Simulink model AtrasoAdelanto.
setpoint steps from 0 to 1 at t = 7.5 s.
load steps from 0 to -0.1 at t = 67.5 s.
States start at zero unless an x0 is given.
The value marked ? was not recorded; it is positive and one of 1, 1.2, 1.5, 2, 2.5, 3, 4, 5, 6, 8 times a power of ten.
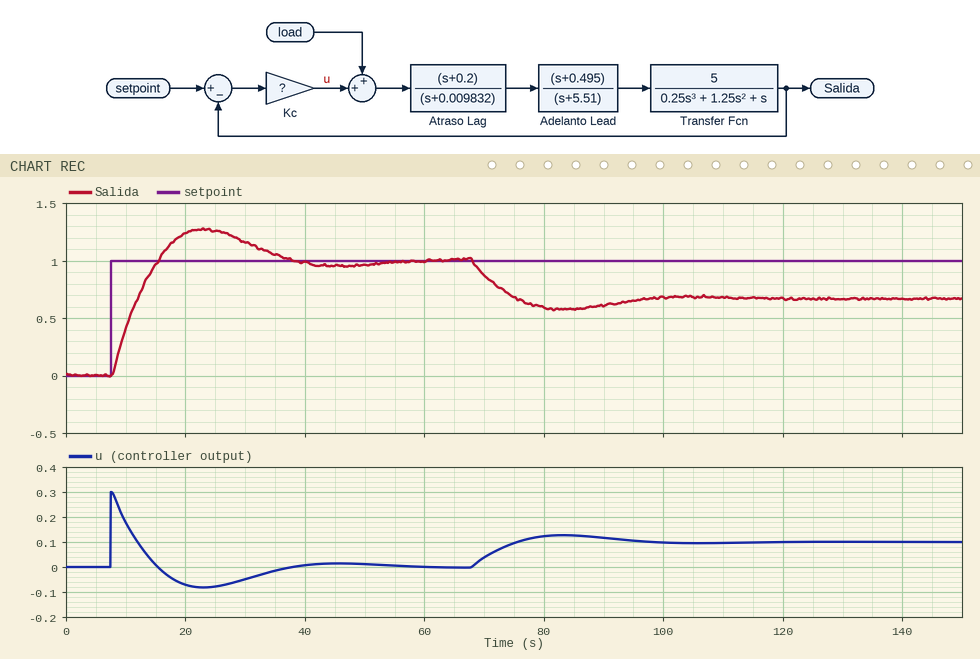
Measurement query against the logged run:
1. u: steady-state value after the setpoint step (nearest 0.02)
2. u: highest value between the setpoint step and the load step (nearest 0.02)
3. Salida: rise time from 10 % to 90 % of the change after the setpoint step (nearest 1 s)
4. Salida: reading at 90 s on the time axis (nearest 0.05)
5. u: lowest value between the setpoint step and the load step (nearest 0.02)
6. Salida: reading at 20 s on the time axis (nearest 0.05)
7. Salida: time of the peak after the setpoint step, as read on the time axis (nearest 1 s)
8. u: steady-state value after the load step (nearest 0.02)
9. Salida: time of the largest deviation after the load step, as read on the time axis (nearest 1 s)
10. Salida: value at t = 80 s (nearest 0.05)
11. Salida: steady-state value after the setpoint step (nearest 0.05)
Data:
0.00
0.30
6 s
0.60
-0.08
1.25
23 s
0.10
83 s
0.60
1.00
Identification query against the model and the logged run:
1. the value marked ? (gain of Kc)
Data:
0.3
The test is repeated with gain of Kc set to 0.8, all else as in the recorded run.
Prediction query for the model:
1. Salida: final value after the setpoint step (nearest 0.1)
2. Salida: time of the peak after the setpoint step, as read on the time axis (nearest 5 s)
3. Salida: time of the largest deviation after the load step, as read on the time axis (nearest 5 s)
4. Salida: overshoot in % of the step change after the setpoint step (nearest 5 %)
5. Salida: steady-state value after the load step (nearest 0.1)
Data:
1.0
15 s
75 s
15 %
0.9
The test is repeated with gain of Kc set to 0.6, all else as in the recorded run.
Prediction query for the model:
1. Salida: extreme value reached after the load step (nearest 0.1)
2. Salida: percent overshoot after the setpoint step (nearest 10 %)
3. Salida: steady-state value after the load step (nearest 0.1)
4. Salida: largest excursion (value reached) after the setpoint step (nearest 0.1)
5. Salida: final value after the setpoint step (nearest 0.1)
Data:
0.8
20 %
0.8
1.2
1.0
